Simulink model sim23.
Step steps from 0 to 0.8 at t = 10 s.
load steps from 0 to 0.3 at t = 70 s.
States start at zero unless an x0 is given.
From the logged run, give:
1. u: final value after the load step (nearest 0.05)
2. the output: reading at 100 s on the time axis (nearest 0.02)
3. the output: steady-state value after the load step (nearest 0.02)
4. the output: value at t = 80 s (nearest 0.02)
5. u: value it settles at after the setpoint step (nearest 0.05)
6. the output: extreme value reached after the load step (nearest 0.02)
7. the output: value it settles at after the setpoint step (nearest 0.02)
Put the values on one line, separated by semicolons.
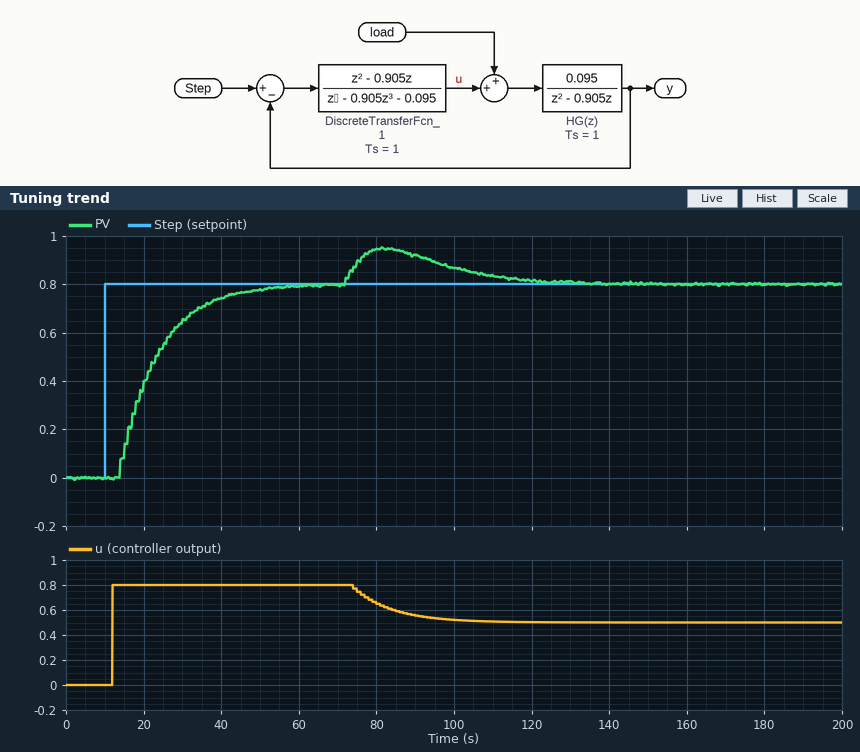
0.50; 0.86; 0.80; 0.94; 0.80; 0.94; 0.80
